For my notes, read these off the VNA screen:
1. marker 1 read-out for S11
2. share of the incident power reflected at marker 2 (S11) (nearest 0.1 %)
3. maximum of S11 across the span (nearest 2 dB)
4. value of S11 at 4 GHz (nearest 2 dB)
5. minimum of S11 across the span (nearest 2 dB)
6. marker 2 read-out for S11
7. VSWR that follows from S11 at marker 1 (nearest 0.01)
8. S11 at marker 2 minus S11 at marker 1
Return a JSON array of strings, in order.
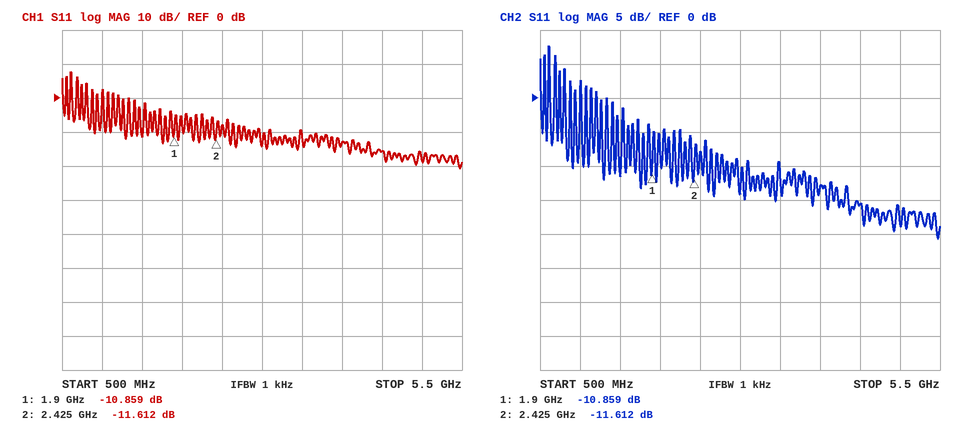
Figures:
["-10.859 dB", "6.9 %", "8 dB", "-14 dB", "-20 dB", "-11.612 dB", "1.80", "-0.753 dB"]
